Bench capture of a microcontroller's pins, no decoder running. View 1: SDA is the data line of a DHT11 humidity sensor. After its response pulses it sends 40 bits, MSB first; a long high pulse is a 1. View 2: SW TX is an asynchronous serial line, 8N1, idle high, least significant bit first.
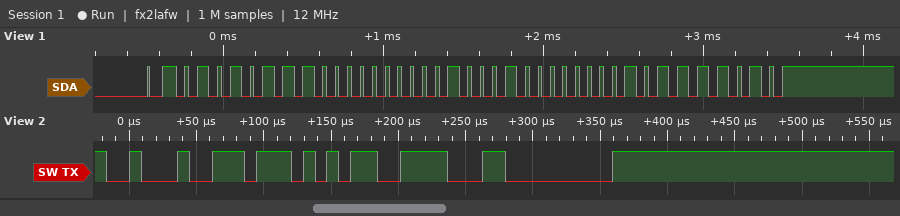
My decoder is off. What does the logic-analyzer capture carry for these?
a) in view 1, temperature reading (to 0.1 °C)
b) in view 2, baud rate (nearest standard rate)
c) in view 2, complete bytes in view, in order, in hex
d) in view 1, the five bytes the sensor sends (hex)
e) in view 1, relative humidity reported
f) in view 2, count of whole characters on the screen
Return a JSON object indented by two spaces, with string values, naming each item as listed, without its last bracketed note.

{
  "in view 1, temperature reading": "34.1 °C",
  "in view 2, baud rate": "115200 baud",
  "in view 2, complete bytes in view, in order, in hex": "0x22 0x57 0x1E 0x00",
  "in view 1, the five bytes the sensor sends": "57 00 22 01 7A",
  "in view 1, relative humidity reported": "87 %",
  "in view 2, count of whole characters on the screen": "4"
}
